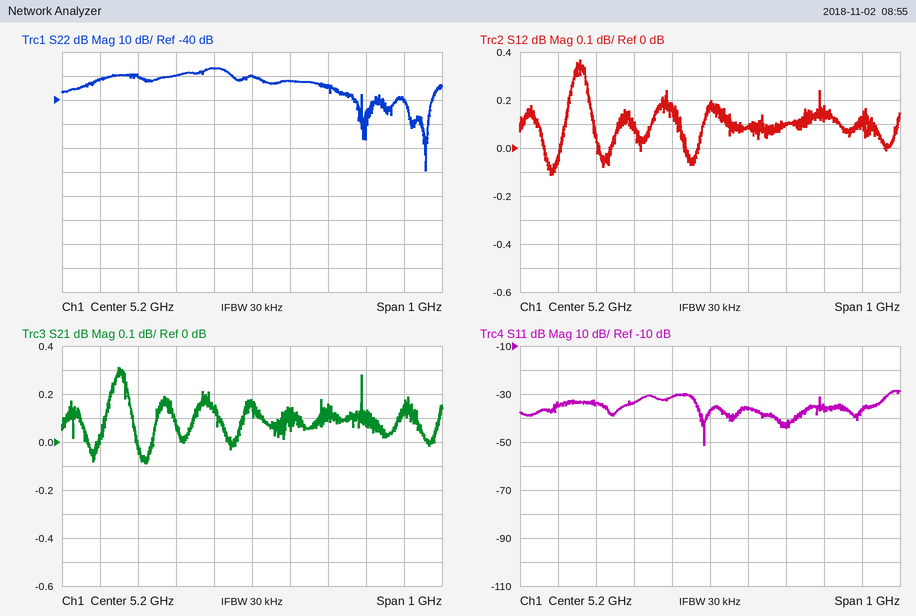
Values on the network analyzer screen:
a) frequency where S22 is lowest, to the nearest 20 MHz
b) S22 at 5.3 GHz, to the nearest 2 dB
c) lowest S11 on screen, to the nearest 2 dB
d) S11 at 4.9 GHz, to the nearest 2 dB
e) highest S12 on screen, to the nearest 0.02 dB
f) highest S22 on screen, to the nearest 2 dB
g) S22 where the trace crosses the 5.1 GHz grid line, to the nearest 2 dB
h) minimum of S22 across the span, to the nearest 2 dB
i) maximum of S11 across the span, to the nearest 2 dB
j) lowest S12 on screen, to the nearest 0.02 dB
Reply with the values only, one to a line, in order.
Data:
5.66 GHz
-32 dB
-52 dB
-34 dB
0.36 dB
-26 dB
-26 dB
-70 dB
-28 dB
-0.12 dB
